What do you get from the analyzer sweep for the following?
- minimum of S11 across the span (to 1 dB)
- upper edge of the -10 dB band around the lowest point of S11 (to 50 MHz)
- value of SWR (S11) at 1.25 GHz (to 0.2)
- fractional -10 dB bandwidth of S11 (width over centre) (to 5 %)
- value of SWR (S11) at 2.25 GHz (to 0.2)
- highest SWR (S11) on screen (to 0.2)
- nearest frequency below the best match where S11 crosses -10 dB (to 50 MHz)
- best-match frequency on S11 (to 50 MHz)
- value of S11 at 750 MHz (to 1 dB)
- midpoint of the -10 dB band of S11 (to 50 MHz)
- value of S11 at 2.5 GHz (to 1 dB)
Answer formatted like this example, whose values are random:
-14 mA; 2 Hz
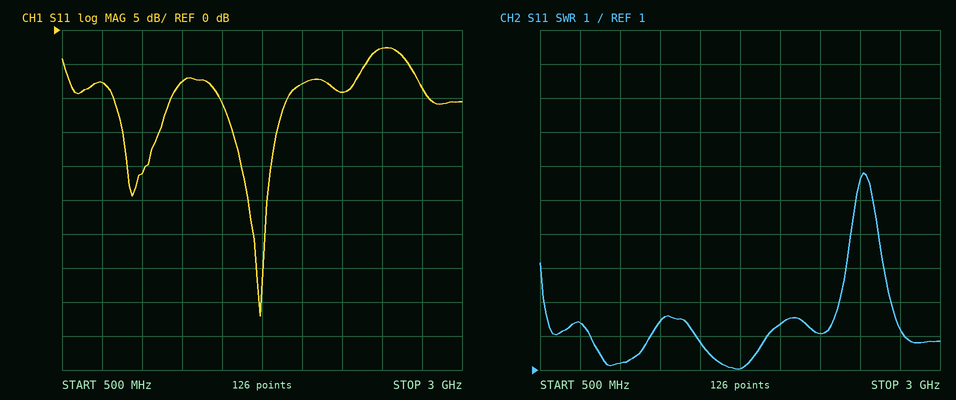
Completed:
-42 dB; 1.90 GHz; 2.4; 25 %; 2.0; 6.8; 1.50 GHz; 1.75 GHz; -8 dB; 1.70 GHz; -3 dB
